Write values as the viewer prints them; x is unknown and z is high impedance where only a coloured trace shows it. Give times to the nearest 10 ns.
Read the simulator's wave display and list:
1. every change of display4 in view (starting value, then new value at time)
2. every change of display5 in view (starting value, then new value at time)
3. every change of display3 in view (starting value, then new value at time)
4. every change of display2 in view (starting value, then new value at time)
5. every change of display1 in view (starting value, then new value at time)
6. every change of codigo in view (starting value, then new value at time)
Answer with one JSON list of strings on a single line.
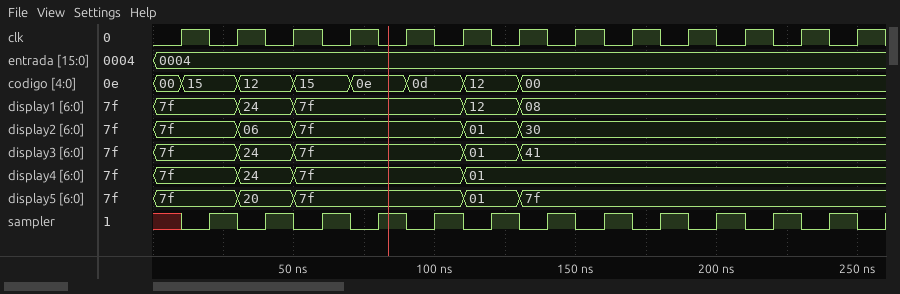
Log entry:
["7f, 24 at 30 ns, 7f at 50 ns, 01 at 110 ns", "7f, 20 at 30 ns, 7f at 50 ns, 01 at 110 ns, 7f at 130 ns", "7f, 24 at 30 ns, 7f at 50 ns, 01 at 110 ns, 41 at 130 ns", "7f, 06 at 30 ns, 7f at 50 ns, 01 at 110 ns, 30 at 130 ns", "7f, 24 at 30 ns, 7f at 50 ns, 12 at 110 ns, 08 at 130 ns", "00, 15 at 10 ns, 12 at 30 ns, 15 at 50 ns, 0e at 70 ns, 0d at 90 ns, 12 at 110 ns, 00 at 130 ns"]
